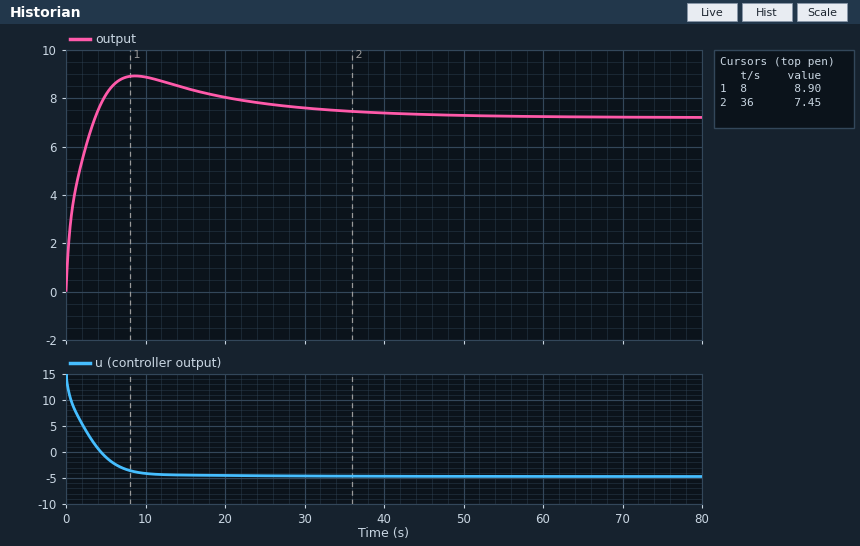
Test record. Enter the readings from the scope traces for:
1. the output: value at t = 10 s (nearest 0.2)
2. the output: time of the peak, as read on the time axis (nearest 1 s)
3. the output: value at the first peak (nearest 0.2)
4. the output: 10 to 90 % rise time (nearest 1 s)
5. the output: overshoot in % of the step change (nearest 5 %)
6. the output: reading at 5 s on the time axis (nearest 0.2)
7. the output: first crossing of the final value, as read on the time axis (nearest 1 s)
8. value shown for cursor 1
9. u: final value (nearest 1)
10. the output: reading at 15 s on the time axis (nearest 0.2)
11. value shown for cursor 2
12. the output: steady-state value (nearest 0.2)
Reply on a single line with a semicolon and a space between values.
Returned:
8.8; 9 s; 9.0; 3 s; 25 %; 8.2; 4 s; 8.90; -5; 8.4; 7.45; 7.2
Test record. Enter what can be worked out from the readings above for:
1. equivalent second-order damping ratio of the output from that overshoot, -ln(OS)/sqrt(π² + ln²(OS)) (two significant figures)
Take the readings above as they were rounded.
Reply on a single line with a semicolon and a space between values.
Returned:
0.40
